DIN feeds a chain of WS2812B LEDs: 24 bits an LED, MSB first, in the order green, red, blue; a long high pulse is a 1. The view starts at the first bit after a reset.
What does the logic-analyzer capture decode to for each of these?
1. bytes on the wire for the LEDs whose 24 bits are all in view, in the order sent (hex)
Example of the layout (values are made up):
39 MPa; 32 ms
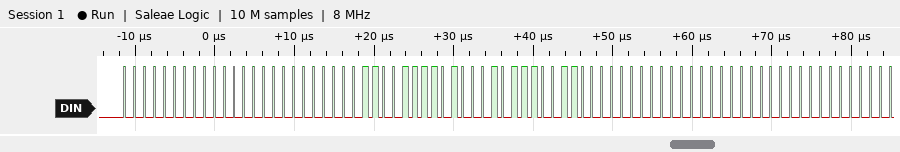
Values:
00 00 00 CF 45 CC 00 00 00
